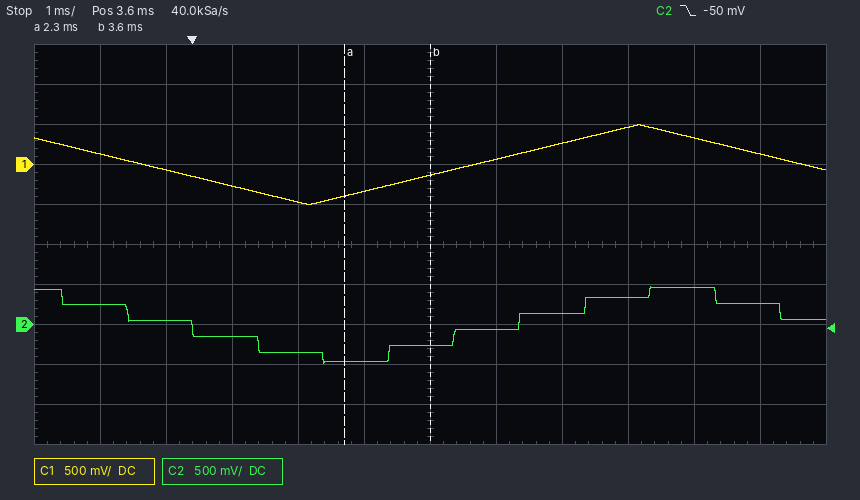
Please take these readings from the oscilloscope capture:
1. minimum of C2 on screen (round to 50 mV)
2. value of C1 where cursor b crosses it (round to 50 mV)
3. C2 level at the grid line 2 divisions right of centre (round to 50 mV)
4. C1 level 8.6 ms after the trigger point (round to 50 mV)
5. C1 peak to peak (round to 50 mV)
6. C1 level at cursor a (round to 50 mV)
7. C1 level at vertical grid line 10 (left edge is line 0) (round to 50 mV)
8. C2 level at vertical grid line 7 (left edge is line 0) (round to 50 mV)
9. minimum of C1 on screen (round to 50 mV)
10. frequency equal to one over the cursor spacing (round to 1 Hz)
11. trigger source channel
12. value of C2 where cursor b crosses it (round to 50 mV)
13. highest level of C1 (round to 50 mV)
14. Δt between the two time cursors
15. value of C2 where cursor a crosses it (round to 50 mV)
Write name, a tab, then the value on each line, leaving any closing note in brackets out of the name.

minimum of C2 on screen	-500 mV
value of C1 where cursor b crosses it	-150 mV
C2 level at the grid line 2 divisions right of centre	150 mV
C1 level 8.6 ms after the trigger point	150 mV
C1 peak to peak	1.00 V
C1 level at cursor a	-400 mV
C1 level at vertical grid line 10 (left edge is line 0)	350 mV
C2 level at vertical grid line 7 (left edge is line 0)	-50 mV
minimum of C1 on screen	-500 mV
frequency equal to one over the cursor spacing	769 Hz
trigger source channel	C2
value of C2 where cursor b crosses it	-250 mV
highest level of C1	500 mV
Δt between the two time cursors	1.3 ms
value of C2 where cursor a crosses it	-450 mV
